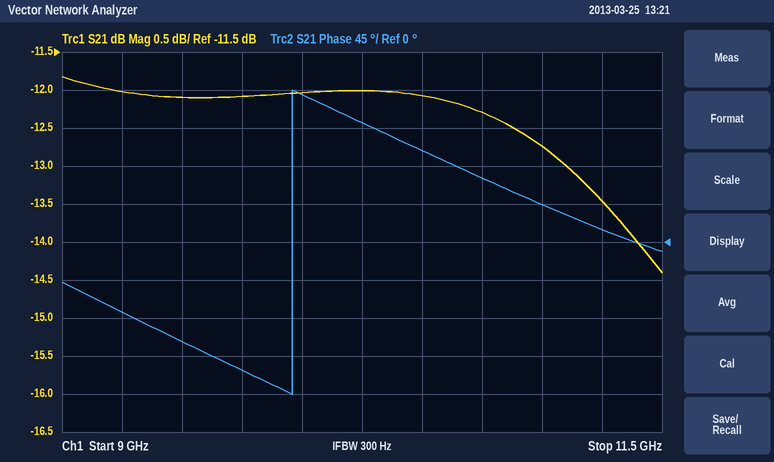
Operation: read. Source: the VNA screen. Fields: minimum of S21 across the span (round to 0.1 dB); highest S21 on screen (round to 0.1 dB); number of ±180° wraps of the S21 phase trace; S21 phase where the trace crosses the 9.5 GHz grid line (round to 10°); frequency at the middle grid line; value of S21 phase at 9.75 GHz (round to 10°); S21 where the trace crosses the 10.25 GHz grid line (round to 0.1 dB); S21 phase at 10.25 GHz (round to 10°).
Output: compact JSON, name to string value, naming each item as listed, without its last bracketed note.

{"minimum of S21 across the span": "-14.4 dB", "highest S21 on screen": "-11.8 dB", "number of ±180° wraps of the S21 phase trace": "1", "S21 phase where the trace crosses the 9.5 GHz grid line": "-120°", "frequency at the middle grid line": "10.25 GHz", "value of S21 phase at 9.75 GHz": "-150°", "S21 where the trace crosses the 10.25 GHz grid line": "-12.0 dB", "S21 phase at 10.25 GHz": "140°"}
